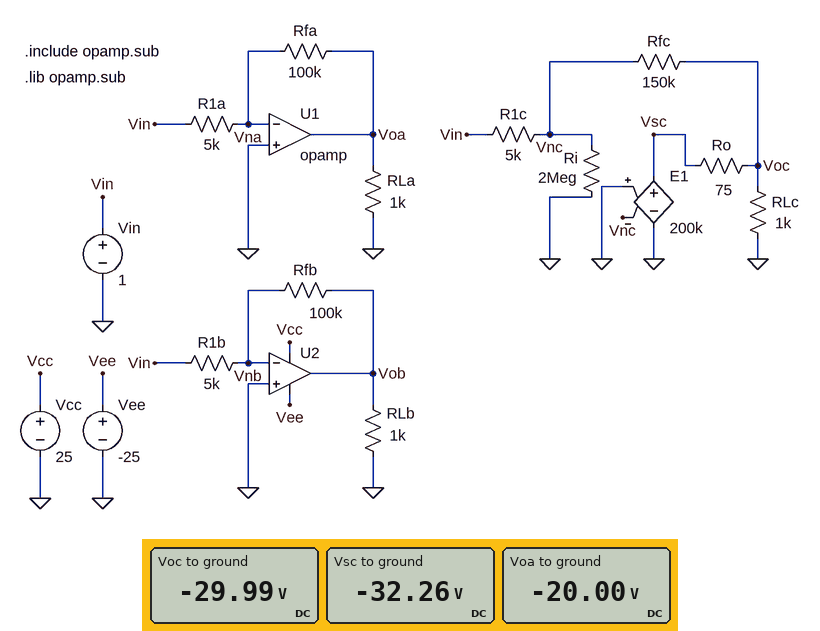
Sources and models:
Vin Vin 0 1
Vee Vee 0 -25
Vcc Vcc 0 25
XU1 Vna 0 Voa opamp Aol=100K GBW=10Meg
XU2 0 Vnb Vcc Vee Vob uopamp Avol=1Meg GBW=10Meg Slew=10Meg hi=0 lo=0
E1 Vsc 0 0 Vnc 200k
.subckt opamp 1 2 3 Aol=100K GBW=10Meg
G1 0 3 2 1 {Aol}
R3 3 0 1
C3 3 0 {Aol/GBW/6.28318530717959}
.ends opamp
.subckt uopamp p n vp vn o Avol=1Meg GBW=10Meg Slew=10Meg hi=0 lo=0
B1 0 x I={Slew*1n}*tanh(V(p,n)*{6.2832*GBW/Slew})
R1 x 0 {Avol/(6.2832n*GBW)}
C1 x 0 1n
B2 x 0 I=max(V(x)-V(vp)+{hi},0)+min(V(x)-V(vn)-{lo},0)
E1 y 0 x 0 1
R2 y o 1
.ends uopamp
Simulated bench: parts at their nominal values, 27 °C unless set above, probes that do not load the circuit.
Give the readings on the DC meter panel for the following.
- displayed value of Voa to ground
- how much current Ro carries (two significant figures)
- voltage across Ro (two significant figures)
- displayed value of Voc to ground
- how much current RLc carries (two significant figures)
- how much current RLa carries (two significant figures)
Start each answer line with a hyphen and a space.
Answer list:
- -20.00 V
- 30 mA
- 2.3 V
- -29.99 V
- 30 mA
- 20 mA
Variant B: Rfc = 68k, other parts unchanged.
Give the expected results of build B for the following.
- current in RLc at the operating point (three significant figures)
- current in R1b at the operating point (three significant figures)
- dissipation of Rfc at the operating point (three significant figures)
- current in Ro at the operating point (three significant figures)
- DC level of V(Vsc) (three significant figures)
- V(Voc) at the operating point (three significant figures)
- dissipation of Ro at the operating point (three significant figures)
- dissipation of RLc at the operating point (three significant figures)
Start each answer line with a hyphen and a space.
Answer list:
- 13.6 mA
- 200 µA
- 2.72 mW
- 13.8 mA
- -14.6 V
- -13.6 V
- 14.3 mW
- 185 mW
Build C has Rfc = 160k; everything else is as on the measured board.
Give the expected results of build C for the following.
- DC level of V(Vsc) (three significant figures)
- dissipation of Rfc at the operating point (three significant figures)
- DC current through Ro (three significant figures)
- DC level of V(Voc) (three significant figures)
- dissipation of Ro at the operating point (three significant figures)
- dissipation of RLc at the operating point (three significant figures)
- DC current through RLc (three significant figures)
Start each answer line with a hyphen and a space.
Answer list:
- -34.4 V
- 6.40 mW
- 32.2 mA
- -32.0 V
- 77.7 mW
- 1.02 W
- 32.0 mA
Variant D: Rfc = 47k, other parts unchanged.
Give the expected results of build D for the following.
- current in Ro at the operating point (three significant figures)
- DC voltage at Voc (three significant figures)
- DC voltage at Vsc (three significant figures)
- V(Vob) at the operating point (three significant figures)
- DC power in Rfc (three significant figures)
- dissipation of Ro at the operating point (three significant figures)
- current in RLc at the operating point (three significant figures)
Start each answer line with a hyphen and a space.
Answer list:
- 9.60 mA
- -9.40 V
- -10.1 V
- -20.0 V
- 1.88 mW
- 6.91 mW
- 9.40 mA
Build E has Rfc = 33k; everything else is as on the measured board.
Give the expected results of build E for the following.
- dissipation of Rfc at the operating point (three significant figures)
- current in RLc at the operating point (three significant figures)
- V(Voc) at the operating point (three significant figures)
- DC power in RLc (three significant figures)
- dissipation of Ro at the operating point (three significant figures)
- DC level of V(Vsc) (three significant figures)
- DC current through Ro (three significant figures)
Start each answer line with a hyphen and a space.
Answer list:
- 1.32 mW
- 6.60 mA
- -6.60 V
- 43.6 mW
- 3.47 mW
- -7.11 V
- 6.80 mA
